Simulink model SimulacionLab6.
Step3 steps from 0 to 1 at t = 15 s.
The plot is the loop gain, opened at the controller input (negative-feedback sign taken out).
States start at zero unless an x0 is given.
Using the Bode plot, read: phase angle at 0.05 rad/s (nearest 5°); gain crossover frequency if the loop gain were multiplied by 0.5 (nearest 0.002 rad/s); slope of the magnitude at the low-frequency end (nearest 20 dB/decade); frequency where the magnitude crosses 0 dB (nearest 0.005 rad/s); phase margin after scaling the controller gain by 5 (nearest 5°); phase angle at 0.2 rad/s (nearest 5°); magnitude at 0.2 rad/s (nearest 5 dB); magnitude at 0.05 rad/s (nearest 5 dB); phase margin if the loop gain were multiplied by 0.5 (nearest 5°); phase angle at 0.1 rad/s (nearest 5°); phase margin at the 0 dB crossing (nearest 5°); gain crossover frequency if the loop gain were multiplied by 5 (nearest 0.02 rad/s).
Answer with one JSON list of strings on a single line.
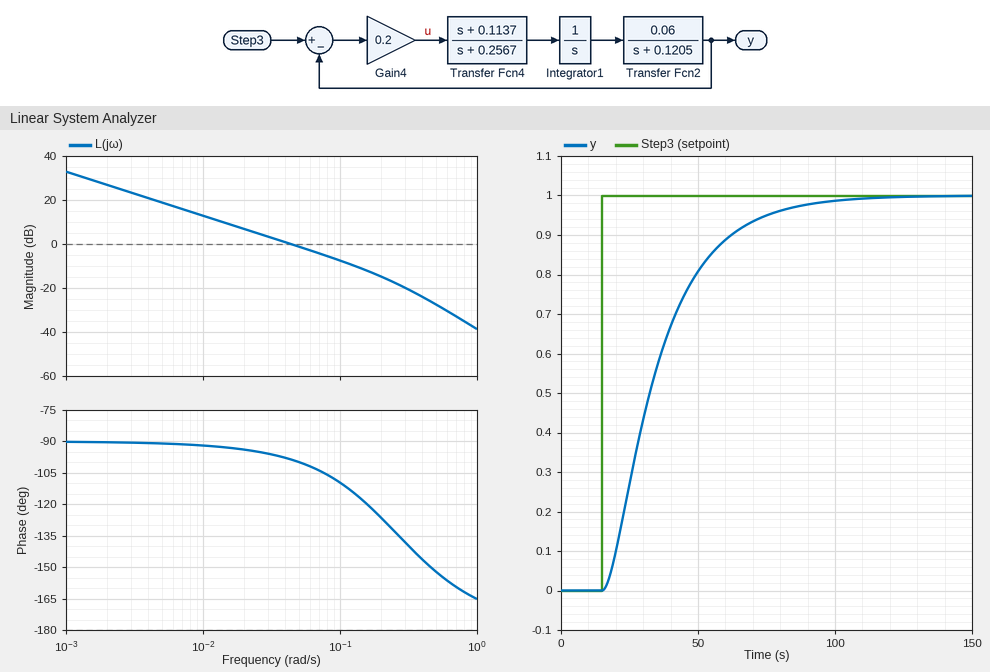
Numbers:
["-100°", "0.022 rad/s", "-20 dB/decade", "0.045 rad/s", "55°", "-125°", "-15 dB", "0 dB", "85°", "-110°", "80°", "0.18 rad/s"]
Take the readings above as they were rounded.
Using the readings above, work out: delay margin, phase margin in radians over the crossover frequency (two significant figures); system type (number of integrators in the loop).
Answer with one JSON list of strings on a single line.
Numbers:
["31 s", "1"]
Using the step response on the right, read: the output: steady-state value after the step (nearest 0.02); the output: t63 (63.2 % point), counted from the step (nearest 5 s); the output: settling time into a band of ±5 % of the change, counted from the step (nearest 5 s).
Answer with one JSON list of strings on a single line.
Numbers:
["1.00", "25 s", "60 s"]
